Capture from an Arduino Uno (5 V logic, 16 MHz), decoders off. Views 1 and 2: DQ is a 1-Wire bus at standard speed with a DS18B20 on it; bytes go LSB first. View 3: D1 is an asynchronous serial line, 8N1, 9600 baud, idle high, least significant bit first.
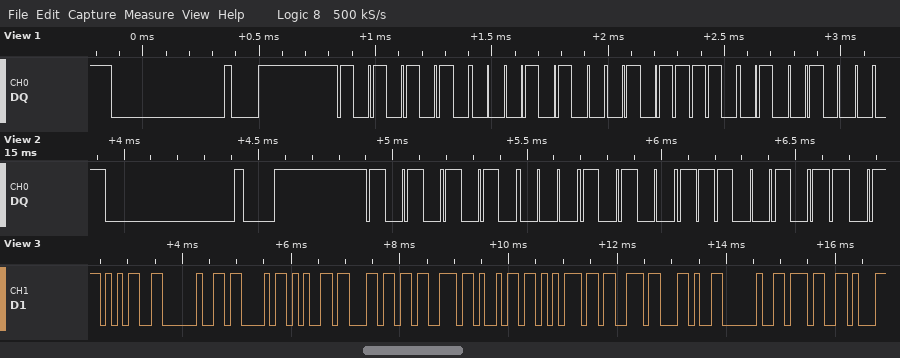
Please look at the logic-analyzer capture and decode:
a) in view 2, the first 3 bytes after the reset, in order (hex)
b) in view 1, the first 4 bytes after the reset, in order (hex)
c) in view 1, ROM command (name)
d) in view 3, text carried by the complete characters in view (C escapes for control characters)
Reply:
55 28 A7
55 28 7A 12
Match ROM
"5 Celsius, 7"
